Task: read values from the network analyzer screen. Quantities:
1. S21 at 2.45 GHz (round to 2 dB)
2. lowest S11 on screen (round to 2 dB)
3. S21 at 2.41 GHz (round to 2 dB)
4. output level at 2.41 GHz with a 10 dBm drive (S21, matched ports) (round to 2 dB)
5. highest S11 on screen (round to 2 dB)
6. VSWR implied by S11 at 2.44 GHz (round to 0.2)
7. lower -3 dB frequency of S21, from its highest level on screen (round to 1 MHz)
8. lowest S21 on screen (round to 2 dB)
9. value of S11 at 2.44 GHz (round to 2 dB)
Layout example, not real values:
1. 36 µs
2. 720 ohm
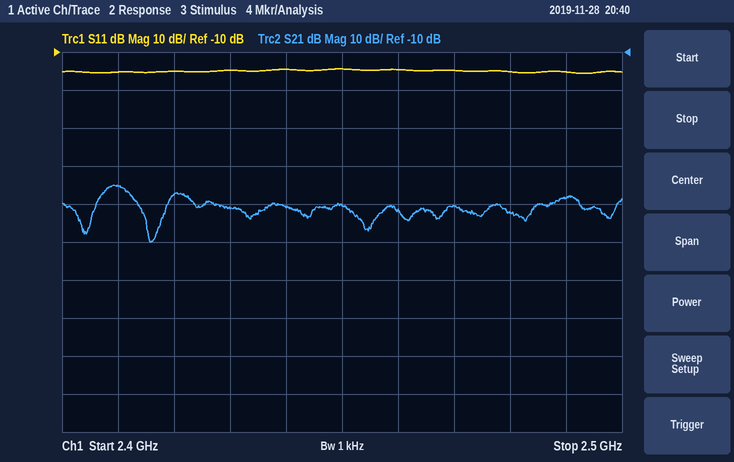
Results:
1. -50 dB
2. -16 dB
3. -46 dB
4. -36 dBm
5. -14 dB
6. 1.4
7. 2.407 GHz
8. -60 dB
9. -14 dB
